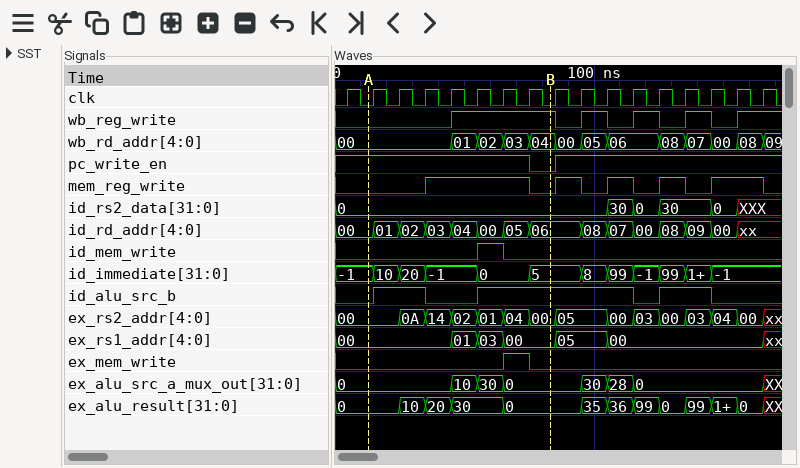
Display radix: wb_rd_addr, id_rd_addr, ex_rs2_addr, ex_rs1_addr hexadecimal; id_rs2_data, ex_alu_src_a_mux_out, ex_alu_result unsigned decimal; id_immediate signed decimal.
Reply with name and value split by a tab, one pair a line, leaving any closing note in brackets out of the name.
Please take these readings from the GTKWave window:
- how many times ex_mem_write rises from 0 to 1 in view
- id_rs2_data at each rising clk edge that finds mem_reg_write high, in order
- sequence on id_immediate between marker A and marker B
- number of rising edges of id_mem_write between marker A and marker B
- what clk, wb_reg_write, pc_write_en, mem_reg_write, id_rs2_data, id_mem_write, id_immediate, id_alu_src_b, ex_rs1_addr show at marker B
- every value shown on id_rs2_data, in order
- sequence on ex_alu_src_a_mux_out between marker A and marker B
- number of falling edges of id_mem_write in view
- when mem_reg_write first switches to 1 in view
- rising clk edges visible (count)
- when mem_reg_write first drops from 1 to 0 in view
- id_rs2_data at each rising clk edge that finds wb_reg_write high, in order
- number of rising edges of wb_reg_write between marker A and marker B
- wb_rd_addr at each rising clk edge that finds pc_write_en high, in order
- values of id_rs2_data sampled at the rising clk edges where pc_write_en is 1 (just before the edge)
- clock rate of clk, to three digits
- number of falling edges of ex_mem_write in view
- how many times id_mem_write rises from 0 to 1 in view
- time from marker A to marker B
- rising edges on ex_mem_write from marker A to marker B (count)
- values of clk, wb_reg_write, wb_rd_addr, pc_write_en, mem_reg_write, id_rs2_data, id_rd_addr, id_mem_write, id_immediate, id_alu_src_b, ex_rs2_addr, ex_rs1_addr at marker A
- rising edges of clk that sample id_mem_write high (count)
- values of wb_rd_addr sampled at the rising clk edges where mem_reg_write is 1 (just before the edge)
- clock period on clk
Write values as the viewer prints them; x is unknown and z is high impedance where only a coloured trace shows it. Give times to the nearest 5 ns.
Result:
how many times ex_mem_write rises from 0 to 1 in view	1
id_rs2_data at each rising clk edge that finds mem_reg_write high, in order	0, 0, 0, 0, 0, 30, 30, 0, XXX
sequence on id_immediate between marker A and marker B	-1, 10, 20, -1, 0, 5
number of rising edges of id_mem_write between marker A and marker B	1
what clk, wb_reg_write, pc_write_en, mem_reg_write, id_rs2_data, id_mem_write, id_immediate, id_alu_src_b, ex_rs1_addr show at marker B	clk=0, wb_reg_write=1, pc_write_en=0, mem_reg_write=0, id_rs2_data=0, id_mem_write=0, id_immediate=5, id_alu_src_b=1, ex_rs1_addr=00
every value shown on id_rs2_data, in order	0, 30, 0, 30, 0, XXX
sequence on ex_alu_src_a_mux_out between marker A and marker B	0, 10, 30, 0
number of falling edges of id_mem_write in view	1
when mem_reg_write first switches to 1 in view	35 ns
rising clk edges visible	17
when mem_reg_write first drops from 1 to 0 in view	75 ns
id_rs2_data at each rising clk edge that finds wb_reg_write high, in order	0, 0, 0, 0, 0, 0, 30, XXX
number of rising edges of wb_reg_write between marker A and marker B	1
wb_rd_addr at each rising clk edge that finds pc_write_en high, in order	00, 00, 00, 00, 00, 01, 02, 03, 00, 05, 06, 06, 08, 07, 00, 08
values of id_rs2_data sampled at the rising clk edges where pc_write_en is 1	0, 0, 0, 0, 0, 0, 0, 0, 0, 0, 30, 0, 30, 30, 0, XXX
clock rate of clk, to three digits	100 MHz
number of falling edges of ex_mem_write in view	1
how many times id_mem_write rises from 0 to 1 in view	1
time from marker A to marker B	70 ns
rising edges on ex_mem_write from marker A to marker B	1
values of clk, wb_reg_write, wb_rd_addr, pc_write_en, mem_reg_write, id_rs2_data, id_rd_addr, id_mem_write, id_immediate, id_alu_src_b, ex_rs2_addr, ex_rs1_addr at marker A	clk=0, wb_reg_write=0, wb_rd_addr=00, pc_write_en=1, mem_reg_write=0, id_rs2_data=0, id_rd_addr=00, id_mem_write=0, id_immediate=-1, id_alu_src_b=0, ex_rs2_addr=00, ex_rs1_addr=00
rising edges of clk that sample id_mem_write high	1
values of wb_rd_addr sampled at the rising clk edges where mem_reg_write is 1	00, 01, 02, 03, 00, 06, 08, 00, 08
clock period on clk	10 ns
